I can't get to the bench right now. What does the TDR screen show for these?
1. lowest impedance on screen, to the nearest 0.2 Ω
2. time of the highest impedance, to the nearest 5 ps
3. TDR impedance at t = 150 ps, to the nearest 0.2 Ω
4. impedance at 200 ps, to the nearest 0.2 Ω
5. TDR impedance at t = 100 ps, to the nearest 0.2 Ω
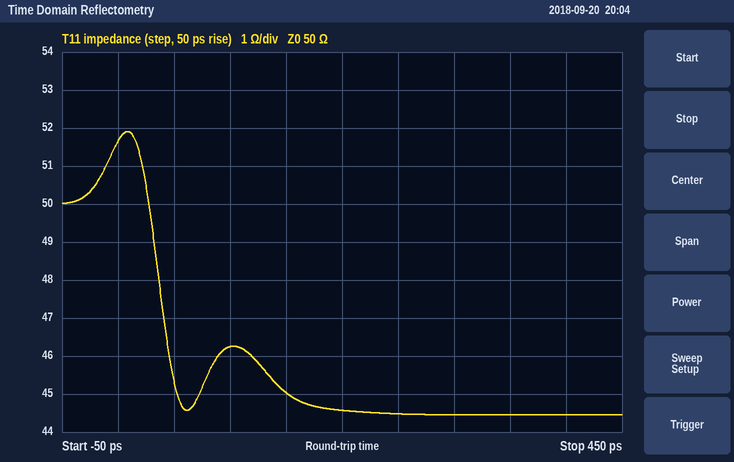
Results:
44.4 Ω
10 ps
45.0 Ω
44.6 Ω
46.2 Ω
